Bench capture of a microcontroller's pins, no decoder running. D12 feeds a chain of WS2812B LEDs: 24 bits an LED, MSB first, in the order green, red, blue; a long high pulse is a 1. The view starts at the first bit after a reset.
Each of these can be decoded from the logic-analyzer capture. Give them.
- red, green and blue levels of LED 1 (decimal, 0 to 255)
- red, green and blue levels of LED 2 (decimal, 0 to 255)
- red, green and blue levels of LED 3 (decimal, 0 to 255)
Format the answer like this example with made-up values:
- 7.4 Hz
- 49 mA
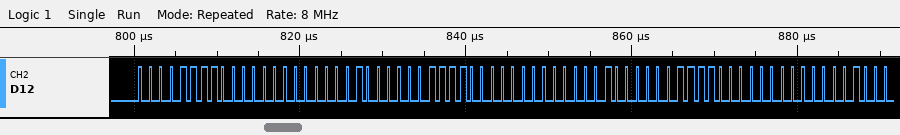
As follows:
- 0, 15, 4
- 0, 15, 4
- 0, 15, 4
